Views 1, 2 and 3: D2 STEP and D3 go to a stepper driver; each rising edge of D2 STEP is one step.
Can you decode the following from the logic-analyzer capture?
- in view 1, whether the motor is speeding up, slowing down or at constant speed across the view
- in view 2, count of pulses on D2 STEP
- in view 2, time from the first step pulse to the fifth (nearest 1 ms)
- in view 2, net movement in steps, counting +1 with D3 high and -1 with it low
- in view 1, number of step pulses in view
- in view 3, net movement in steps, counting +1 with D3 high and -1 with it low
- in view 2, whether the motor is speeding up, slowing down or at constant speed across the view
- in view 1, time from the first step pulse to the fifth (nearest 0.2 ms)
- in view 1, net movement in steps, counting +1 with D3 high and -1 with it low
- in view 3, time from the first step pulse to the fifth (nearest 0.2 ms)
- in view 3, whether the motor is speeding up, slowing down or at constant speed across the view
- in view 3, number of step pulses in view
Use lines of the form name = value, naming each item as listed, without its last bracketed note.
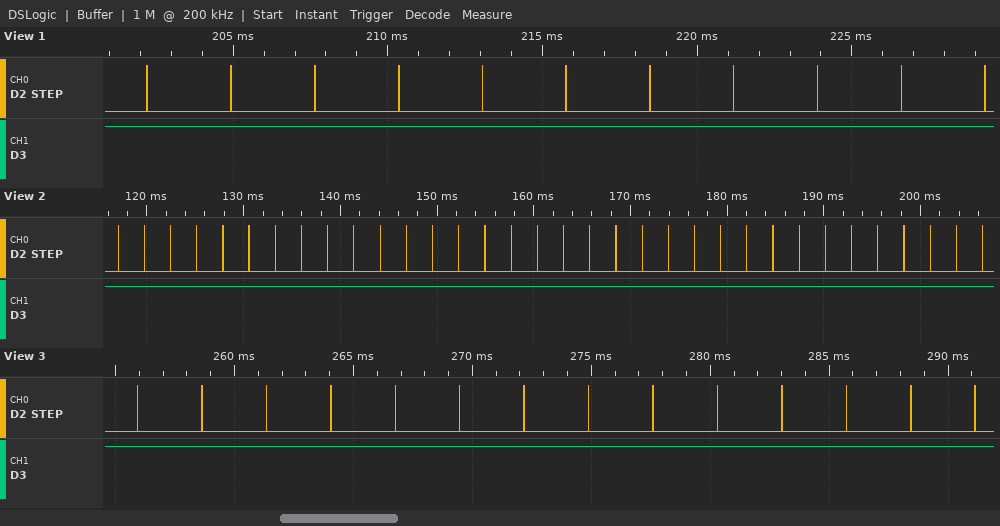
in view 1, whether the motor is speeding up, slowing down or at constant speed across the view = constant speed
in view 2, count of pulses on D2 STEP = 34
in view 2, time from the first step pulse to the fifth = 11 ms
in view 2, net movement in steps, counting +1 with D3 high and -1 with it low = +34
in view 1, number of step pulses in view = 11
in view 3, net movement in steps, counting +1 with D3 high and -1 with it low = +14
in view 2, whether the motor is speeding up, slowing down or at constant speed across the view = constant speed
in view 1, time from the first step pulse to the fifth = 10.8 ms
in view 1, net movement in steps, counting +1 with D3 high and -1 with it low = +11
in view 3, time from the first step pulse to the fifth = 10.8 ms
in view 3, whether the motor is speeding up, slowing down or at constant speed across the view = constant speed
in view 3, number of step pulses in view = 14
